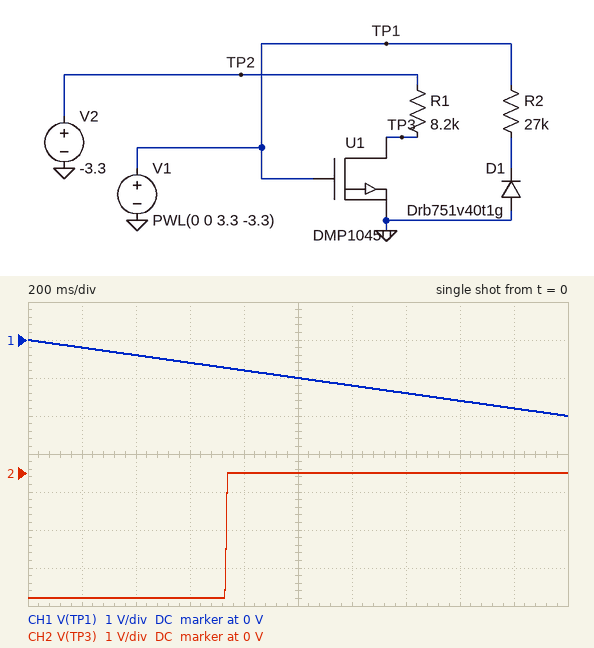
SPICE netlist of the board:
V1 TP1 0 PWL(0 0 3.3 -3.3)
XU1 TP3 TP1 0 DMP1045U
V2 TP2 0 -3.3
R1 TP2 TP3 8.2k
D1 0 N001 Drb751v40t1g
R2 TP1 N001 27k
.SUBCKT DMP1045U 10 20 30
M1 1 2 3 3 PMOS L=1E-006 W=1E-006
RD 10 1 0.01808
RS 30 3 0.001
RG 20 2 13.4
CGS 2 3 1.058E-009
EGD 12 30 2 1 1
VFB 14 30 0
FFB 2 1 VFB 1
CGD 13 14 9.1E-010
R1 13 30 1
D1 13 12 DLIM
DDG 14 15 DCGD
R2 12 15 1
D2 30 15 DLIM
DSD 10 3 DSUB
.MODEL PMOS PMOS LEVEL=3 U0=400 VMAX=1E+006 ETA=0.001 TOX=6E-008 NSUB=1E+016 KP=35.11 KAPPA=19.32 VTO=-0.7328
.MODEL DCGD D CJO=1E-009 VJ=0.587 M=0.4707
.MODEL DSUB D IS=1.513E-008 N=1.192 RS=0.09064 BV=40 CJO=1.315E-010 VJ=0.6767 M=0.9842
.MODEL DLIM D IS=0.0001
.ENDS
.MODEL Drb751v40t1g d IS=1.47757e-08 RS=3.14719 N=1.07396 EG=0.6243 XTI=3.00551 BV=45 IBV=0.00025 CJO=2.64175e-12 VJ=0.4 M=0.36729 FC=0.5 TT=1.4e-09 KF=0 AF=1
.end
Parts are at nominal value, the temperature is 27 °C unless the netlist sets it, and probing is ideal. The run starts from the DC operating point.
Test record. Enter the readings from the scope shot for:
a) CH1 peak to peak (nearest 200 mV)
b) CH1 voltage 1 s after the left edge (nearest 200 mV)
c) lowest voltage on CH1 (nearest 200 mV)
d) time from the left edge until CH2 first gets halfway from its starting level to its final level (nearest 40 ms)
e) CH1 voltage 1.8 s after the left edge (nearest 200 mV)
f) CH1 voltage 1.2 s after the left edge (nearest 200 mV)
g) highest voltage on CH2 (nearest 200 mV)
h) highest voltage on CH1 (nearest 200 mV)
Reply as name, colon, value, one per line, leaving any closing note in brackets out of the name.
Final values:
CH1 peak to peak: 2.0 V
CH1 voltage 1 s after the left edge: -1.0 V
lowest voltage on CH1: -2.0 V
time from the left edge until CH2 first gets halfway from its starting level to its final level: 720 ms
CH1 voltage 1.8 s after the left edge: -1.8 V
CH1 voltage 1.2 s after the left edge: -1.2 V
highest voltage on CH2: 0 V
highest voltage on CH1: 0 V
